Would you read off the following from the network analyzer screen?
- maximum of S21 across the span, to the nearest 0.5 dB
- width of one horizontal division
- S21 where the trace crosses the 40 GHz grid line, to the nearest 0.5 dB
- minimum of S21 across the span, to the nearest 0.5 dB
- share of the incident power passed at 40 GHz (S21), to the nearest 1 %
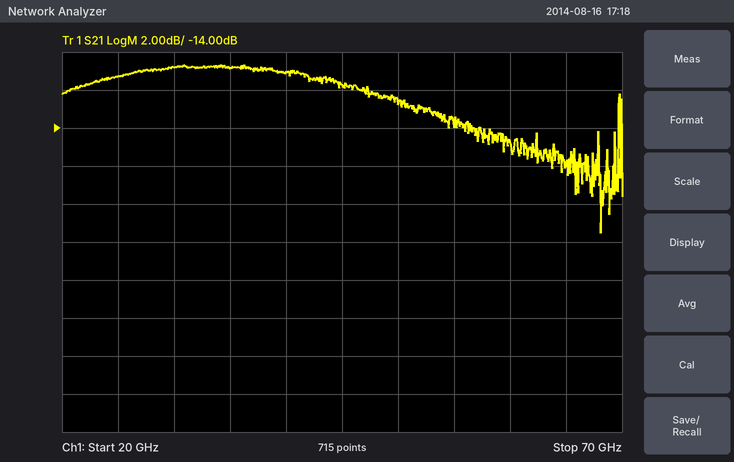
-10.5 dB
5 GHz
-11.0 dB
-19.5 dB
8 %
